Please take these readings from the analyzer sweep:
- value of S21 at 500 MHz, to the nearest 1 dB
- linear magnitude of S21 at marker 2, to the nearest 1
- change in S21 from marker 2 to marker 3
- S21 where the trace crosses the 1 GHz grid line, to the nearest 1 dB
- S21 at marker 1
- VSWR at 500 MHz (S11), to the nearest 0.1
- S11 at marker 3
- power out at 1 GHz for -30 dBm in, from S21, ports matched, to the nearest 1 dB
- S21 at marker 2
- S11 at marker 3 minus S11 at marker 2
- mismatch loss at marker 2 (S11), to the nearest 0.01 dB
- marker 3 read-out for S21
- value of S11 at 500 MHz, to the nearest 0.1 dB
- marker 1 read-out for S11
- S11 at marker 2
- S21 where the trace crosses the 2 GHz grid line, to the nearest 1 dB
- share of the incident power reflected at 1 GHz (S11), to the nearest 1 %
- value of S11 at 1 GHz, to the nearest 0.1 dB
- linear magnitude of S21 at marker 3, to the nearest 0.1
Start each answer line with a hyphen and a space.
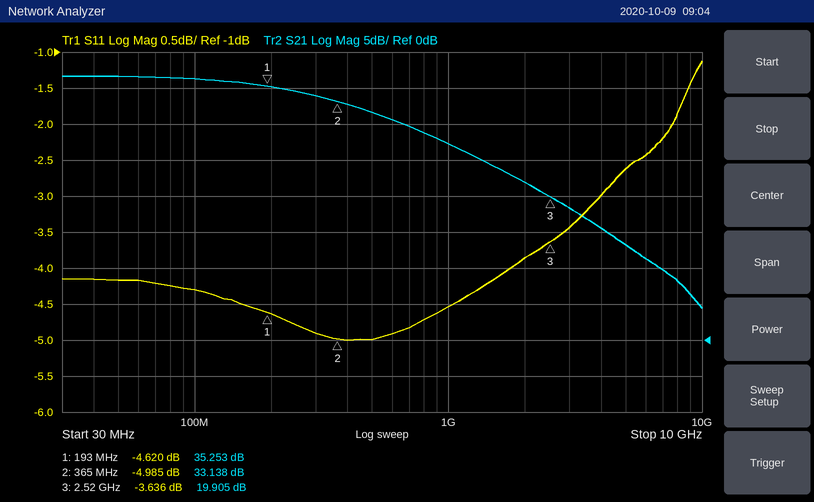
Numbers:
- 32 dB
- 45
- -13.233 dB
- 27 dB
- 35.253 dB
- 3.6
- -3.636 dB
- -3 dBm
- 33.138 dB
- 1.349 dB
- 1.66 dB
- 19.905 dB
- -5.0 dB
- -4.620 dB
- -4.985 dB
- 22 dB
- 35 %
- -4.5 dB
- 9.9
